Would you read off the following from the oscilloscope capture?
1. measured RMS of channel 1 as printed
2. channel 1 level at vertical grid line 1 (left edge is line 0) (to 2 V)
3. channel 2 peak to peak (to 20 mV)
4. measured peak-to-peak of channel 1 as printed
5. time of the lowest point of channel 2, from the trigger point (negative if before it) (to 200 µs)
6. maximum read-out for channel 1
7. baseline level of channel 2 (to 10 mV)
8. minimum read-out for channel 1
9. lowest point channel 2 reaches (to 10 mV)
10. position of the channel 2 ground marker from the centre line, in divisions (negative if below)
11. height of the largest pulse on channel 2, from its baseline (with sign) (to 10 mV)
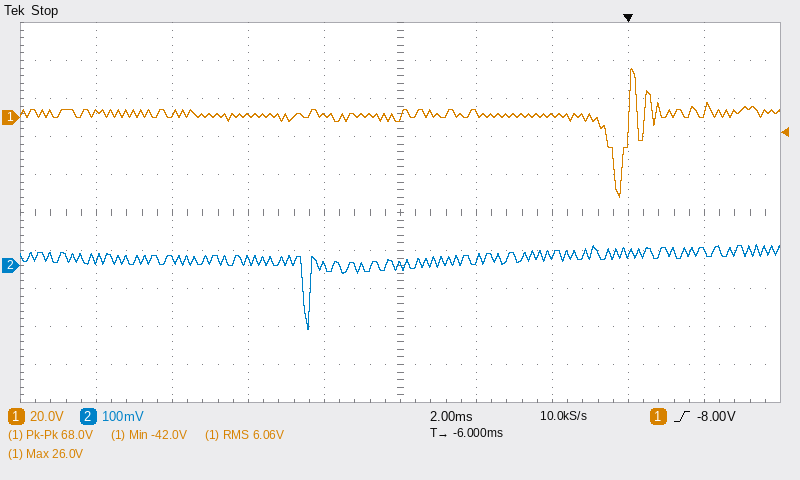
6.06 V
2 V
220 mV
68.0 V
-8.4 ms
26.0 V
20 mV
-42.0 V
-170 mV
-1.4 div
-190 mV
